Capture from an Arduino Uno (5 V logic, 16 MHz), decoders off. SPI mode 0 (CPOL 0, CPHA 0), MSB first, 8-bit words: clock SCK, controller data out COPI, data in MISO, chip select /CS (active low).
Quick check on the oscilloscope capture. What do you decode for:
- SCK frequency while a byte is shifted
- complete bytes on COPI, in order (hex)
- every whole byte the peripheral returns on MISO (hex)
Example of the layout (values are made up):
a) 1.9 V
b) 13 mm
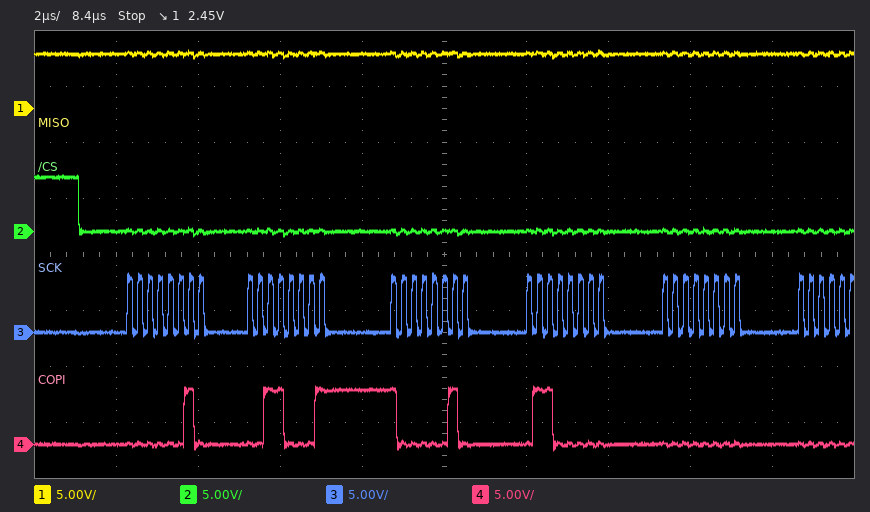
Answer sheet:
a) 4 MHz
b) 02 31 82 60 00
c) FF FF FF FF FF
